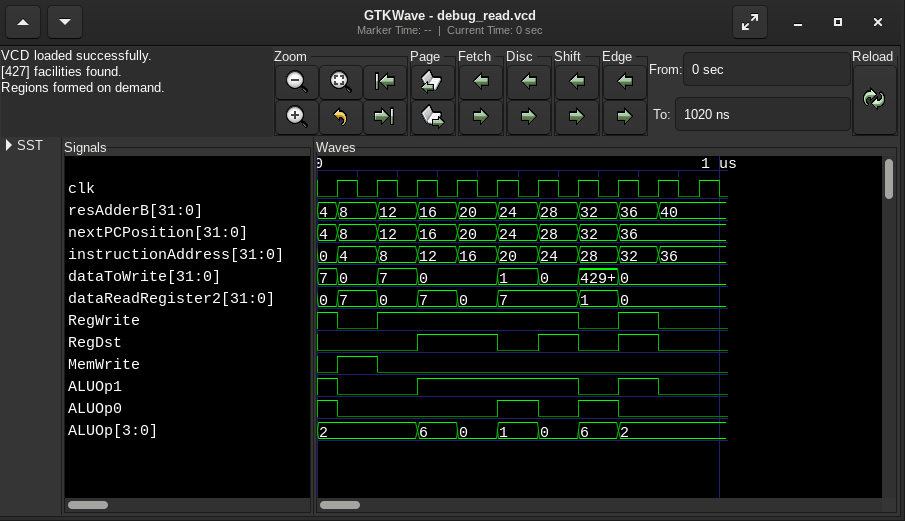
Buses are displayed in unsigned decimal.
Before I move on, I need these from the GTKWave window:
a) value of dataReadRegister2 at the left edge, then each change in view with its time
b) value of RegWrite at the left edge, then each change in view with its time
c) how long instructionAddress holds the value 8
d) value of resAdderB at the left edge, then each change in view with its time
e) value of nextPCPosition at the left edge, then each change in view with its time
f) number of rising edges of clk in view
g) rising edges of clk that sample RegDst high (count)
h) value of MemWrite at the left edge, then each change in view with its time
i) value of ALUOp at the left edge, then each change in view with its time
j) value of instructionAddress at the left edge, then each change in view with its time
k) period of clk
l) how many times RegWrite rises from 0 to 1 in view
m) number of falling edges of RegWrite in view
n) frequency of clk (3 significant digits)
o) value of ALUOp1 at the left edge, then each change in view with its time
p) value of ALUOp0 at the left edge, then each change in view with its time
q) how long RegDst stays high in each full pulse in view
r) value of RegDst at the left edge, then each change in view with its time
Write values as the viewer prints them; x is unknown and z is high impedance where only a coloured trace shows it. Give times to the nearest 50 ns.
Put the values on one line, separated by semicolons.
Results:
0, 7 at 50 ns, 0 at 150 ns, 7 at 250 ns, 0 at 350 ns, 7 at 450 ns, 1 at 650 ns, 0 at 750 ns; 1, 0 at 50 ns, 1 at 150 ns, 0 at 650 ns, 1 at 750 ns, 0 at 850 ns; 100 ns; 4, 8 at 50 ns, 12 at 150 ns, 16 at 250 ns, 20 at 350 ns, 24 at 450 ns, 28 at 550 ns, 32 at 650 ns, 36 at 750 ns, 40 at 850 ns; 4, 8 at 50 ns, 12 at 150 ns, 16 at 250 ns, 20 at 350 ns, 24 at 450 ns, 28 at 550 ns, 32 at 650 ns, 36 at 750 ns; 10; 4; 0, 1 at 50 ns, 0 at 150 ns; 2, 6 at 250 ns, 0 at 350 ns, 1 at 450 ns, 0 at 550 ns, 6 at 650 ns, 2 at 750 ns; 0, 4 at 50 ns, 8 at 150 ns, 12 at 250 ns, 16 at 350 ns, 20 at 450 ns, 24 at 550 ns, 28 at 650 ns, 32 at 750 ns, 36 at 850 ns; 100 ns; 2; 3; 10.0 MHz; 1, 0 at 50 ns, 1 at 250 ns, 0 at 650 ns, 1 at 750 ns, 0 at 850 ns; 1, 0 at 50 ns, 1 at 450 ns, 0 at 550 ns, 1 at 650 ns, 0 at 750 ns; 200 ns, 100 ns, 100 ns; 0, 1 at 250 ns, 0 at 450 ns, 1 at 550 ns, 0 at 650 ns, 1 at 750 ns, 0 at 850 ns
